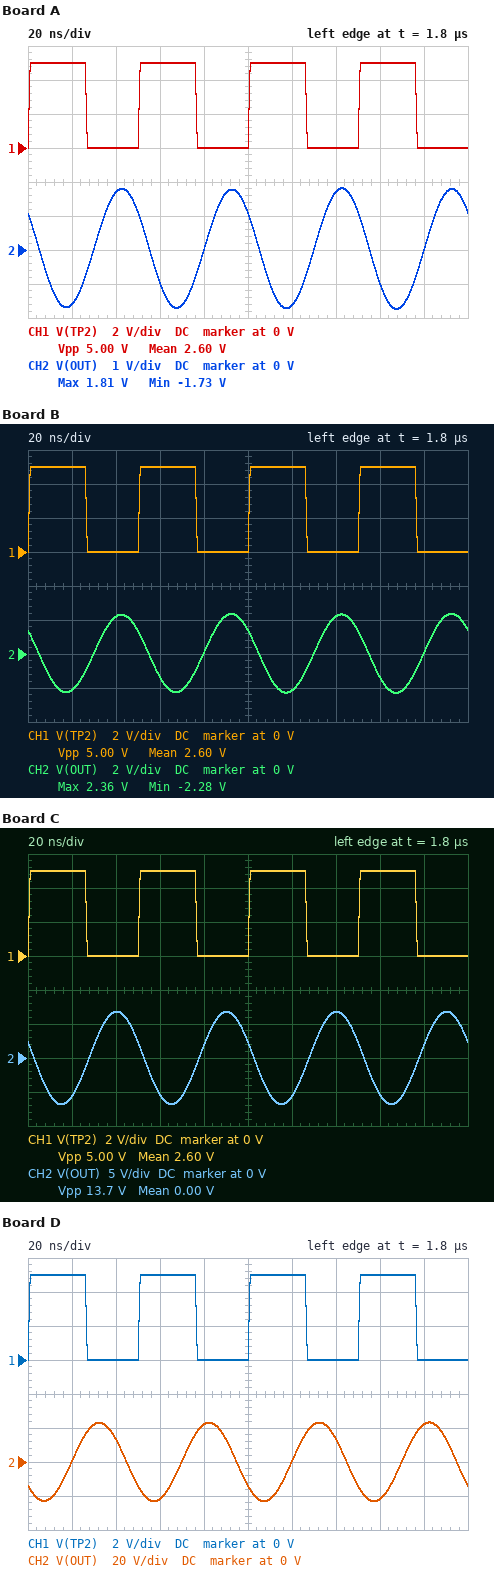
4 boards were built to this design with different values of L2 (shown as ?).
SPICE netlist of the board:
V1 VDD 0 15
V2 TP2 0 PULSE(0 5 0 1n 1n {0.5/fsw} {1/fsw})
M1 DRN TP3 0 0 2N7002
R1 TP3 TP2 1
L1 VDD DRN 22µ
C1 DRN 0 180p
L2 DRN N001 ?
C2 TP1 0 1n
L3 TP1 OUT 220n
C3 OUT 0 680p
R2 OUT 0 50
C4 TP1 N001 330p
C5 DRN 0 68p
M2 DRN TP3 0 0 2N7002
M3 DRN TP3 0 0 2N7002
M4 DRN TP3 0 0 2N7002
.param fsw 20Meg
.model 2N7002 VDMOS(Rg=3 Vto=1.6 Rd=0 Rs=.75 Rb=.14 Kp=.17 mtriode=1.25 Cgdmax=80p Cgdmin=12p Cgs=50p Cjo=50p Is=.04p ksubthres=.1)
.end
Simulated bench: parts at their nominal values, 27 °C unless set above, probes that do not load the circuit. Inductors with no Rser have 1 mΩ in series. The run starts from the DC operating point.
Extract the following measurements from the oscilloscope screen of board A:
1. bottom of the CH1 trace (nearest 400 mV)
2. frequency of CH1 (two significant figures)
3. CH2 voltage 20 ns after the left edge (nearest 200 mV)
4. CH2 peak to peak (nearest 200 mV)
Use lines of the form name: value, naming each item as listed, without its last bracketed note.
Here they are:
bottom of the CH1 trace: 0 V
frequency of CH1: 20 MHz
CH2 voltage 20 ns after the left edge: -1.6 V
CH2 peak to peak: 3.6 V
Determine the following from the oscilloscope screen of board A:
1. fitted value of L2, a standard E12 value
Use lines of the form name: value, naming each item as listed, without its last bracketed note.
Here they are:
fitted value of L2, a standard E12 value: 1.2 µH
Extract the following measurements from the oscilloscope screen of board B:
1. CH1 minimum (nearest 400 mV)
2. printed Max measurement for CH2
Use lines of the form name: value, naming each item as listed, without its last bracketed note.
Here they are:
CH1 minimum: 0 V
printed Max measurement for CH2: 2.36 V
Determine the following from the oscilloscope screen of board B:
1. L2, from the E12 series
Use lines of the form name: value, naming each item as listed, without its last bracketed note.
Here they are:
L2, from the E12 series: 1 µH
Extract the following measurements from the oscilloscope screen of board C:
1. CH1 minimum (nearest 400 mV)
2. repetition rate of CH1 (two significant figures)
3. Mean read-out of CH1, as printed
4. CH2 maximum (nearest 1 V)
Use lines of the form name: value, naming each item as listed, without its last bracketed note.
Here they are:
CH1 minimum: 0 V
repetition rate of CH1: 20 MHz
Mean read-out of CH1, as printed: 2.60 V
CH2 maximum: 7 V
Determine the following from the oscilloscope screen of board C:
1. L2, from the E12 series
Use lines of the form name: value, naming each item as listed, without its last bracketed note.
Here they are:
L2, from the E12 series: 560 nH
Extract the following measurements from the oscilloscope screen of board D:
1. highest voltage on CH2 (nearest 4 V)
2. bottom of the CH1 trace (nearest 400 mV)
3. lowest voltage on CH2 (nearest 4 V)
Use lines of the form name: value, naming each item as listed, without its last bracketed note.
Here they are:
highest voltage on CH2: 24 V
bottom of the CH1 trace: 0 V
lowest voltage on CH2: -24 V
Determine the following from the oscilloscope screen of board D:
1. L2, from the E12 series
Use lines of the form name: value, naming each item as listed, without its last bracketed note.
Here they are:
L2, from the E12 series: 390 nH
